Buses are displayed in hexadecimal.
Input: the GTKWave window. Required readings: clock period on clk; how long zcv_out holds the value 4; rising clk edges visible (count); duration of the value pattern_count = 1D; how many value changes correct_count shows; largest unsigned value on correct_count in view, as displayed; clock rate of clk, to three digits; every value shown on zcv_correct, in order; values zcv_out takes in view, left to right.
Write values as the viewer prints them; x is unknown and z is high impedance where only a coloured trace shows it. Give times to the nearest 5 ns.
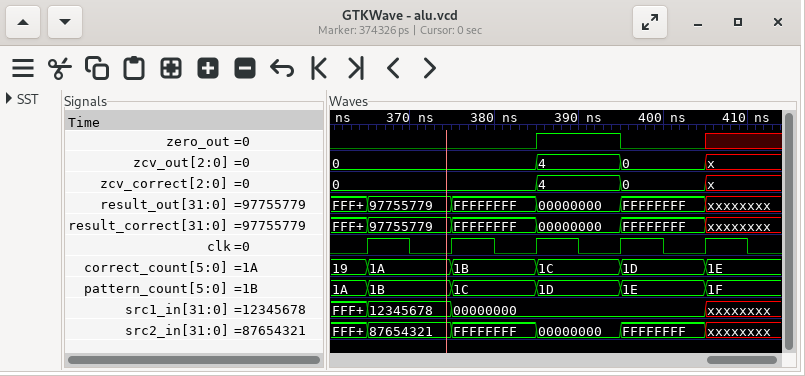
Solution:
10 ns
10 ns
5
10 ns
5
1E
100 MHz
0, 4, 0, x
0, 4, 0, x
